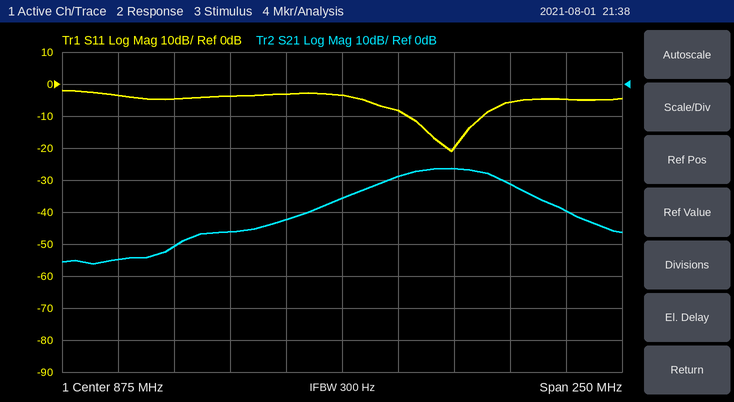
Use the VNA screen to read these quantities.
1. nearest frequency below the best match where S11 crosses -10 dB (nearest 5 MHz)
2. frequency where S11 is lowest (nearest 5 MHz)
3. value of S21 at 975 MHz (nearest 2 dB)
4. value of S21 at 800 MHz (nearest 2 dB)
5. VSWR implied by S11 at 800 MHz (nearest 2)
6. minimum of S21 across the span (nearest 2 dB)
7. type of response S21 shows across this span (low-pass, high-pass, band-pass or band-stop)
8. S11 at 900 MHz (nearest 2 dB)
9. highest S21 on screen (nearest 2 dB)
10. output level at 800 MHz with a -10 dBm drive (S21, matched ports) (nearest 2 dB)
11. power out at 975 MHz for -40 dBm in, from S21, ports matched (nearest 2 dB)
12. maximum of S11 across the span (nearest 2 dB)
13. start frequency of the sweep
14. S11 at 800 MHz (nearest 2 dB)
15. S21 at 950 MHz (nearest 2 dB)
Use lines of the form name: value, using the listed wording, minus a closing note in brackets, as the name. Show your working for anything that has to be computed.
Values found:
nearest frequency below the best match where S11 crosses -10 dB: 905 MHz
frequency where S11 is lowest: 925 MHz
value of S21 at 975 MHz: -40 dB
value of S21 at 800 MHz: -50 dB
VSWR implied by S11 at 800 MHz: |Γ| = 10^(-4/20) = 0.6310; VSWR = (1 + 0.6310)/(1 − 0.6310) ≈ 4
minimum of S21 across the span: -56 dB
type of response S21 shows across this span: band-pass
S11 at 900 MHz: -8 dB
highest S21 on screen: -26 dB
output level at 800 MHz with a -10 dBm drive (S21, matched ports): -10 dBm + (-50 dB) = -60 dBm
power out at 975 MHz for -40 dBm in, from S21, ports matched: -40 dBm + (-40 dB) = -80 dBm
maximum of S11 across the span: -2 dB
start frequency of the sweep: 750 MHz
S11 at 800 MHz: -4 dB
S21 at 950 MHz: -32 dB
